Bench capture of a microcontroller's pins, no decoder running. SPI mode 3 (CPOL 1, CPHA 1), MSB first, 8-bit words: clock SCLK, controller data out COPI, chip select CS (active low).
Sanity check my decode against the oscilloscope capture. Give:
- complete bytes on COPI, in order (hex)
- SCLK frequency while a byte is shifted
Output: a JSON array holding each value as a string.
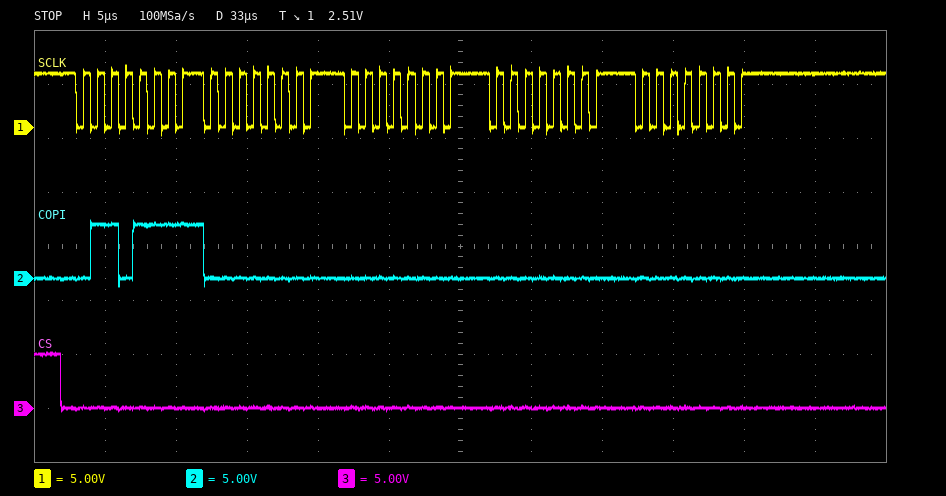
["6F 00 00 00 00", "1 MHz"]
